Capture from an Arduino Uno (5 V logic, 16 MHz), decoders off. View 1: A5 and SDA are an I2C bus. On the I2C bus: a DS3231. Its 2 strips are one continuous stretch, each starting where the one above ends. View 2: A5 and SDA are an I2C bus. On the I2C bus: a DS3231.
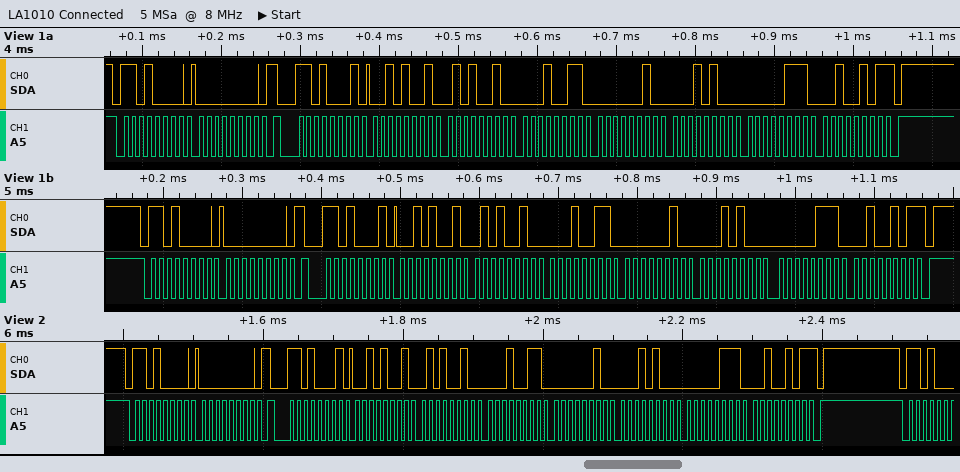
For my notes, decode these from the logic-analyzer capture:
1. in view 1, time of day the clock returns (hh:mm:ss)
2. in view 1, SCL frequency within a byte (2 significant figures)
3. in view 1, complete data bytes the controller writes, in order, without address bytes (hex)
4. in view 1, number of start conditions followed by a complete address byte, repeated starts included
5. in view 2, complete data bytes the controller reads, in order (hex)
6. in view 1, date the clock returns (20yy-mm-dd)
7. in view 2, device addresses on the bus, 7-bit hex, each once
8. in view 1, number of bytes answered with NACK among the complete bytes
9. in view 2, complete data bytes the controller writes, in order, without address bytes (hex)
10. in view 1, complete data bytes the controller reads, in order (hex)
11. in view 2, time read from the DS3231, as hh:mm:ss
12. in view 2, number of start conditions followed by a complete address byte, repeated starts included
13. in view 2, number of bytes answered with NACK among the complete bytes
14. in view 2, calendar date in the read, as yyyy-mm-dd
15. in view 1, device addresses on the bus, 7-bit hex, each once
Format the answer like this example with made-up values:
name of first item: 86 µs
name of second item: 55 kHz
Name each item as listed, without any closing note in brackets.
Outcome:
in view 1, time of day the clock returns: 13:52:29
in view 1, SCL frequency within a byte: 100 kHz
in view 1, complete data bytes the controller writes, in order, without address bytes: 00 00
in view 1, number of start conditions followed by a complete address byte, repeated starts included: 4
in view 2, complete data bytes the controller reads, in order: 29 52 13 02 14 07 25
in view 1, date the clock returns: 2025-07-14
in view 2, device addresses on the bus, 7-bit hex, each once: 0x68
in view 1, number of bytes answered with NACK among the complete bytes: 2
in view 2, complete data bytes the controller writes, in order, without address bytes: 00
in view 1, complete data bytes the controller reads, in order: 29 52 13 02 14 07 25 29 52 13 02 14 07 25
in view 2, time read from the DS3231, as hh:mm:ss: 13:52:29
in view 2, number of start conditions followed by a complete address byte, repeated starts included: 2
in view 2, number of bytes answered with NACK among the complete bytes: 1
in view 2, calendar date in the read, as yyyy-mm-dd: 2025-07-14
in view 1, device addresses on the bus, 7-bit hex, each once: 0x68
